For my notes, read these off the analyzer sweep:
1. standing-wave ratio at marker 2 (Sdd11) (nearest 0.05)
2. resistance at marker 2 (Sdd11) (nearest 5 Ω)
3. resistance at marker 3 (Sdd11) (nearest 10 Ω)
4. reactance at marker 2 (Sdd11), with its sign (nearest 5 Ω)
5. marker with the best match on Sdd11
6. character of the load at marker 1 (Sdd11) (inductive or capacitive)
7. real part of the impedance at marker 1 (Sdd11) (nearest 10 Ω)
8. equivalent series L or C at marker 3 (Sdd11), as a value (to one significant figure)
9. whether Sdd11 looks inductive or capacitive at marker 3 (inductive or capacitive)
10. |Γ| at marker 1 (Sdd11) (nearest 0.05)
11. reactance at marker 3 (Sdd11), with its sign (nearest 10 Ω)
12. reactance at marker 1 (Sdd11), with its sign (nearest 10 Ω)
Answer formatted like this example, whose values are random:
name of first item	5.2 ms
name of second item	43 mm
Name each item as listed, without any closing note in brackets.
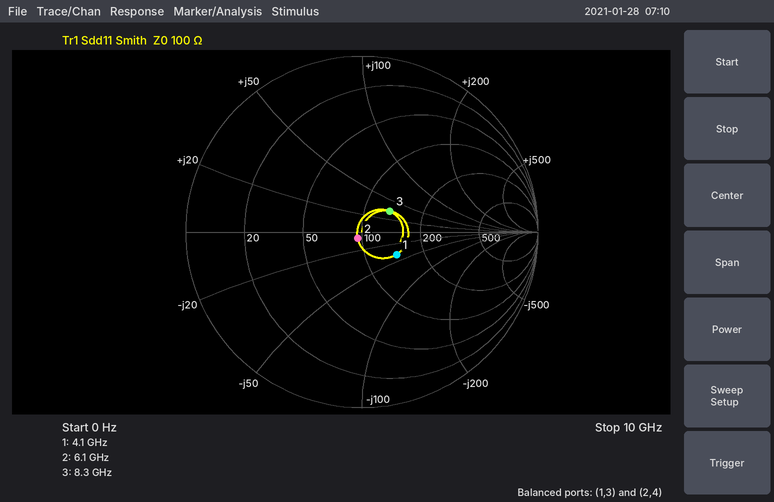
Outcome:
standing-wave ratio at marker 2 (Sdd11)	1.10
resistance at marker 2 (Sdd11)	95 Ω
resistance at marker 3 (Sdd11)	130 Ω
reactance at marker 2 (Sdd11), with its sign	-5 Ω
marker with the best match on Sdd11	marker 2
character of the load at marker 1 (Sdd11)	capacitive
real part of the impedance at marker 1 (Sdd11)	140 Ω
equivalent series L or C at marker 3 (Sdd11), as a value	600 pH
whether Sdd11 looks inductive or capacitive at marker 3	inductive
|Γ| at marker 1 (Sdd11)	0.25
reactance at marker 3 (Sdd11), with its sign	+30 Ω
reactance at marker 1 (Sdd11), with its sign	-40 Ω
